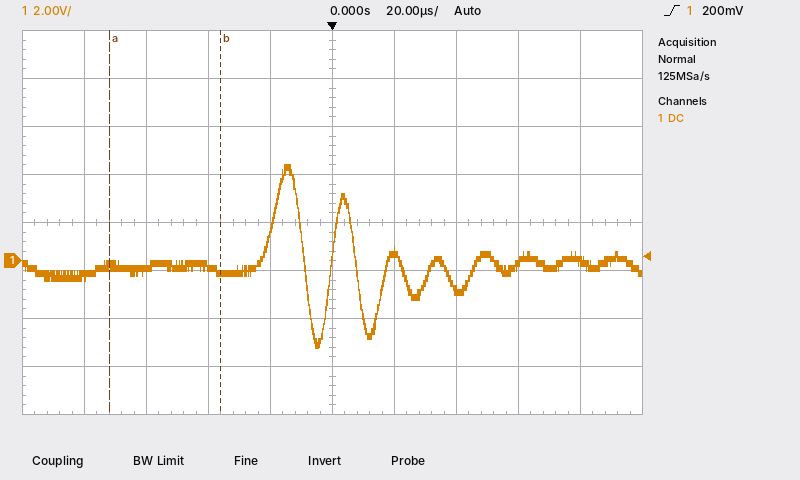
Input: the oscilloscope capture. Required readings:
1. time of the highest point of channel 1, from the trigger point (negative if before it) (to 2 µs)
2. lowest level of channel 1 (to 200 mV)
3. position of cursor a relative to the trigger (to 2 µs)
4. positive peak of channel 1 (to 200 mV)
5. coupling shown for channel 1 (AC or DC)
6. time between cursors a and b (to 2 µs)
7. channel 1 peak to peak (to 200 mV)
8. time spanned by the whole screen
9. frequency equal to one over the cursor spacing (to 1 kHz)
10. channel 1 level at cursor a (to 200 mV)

-14 µs
-3.6 V
-72 µs
4.0 V
DC
36 µs
7.6 V
200 µs
28 kHz
-200 mV
